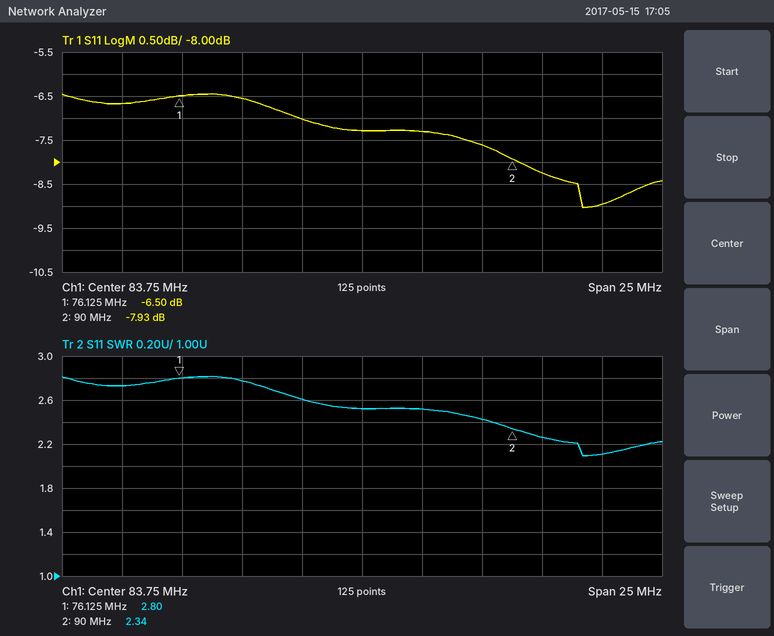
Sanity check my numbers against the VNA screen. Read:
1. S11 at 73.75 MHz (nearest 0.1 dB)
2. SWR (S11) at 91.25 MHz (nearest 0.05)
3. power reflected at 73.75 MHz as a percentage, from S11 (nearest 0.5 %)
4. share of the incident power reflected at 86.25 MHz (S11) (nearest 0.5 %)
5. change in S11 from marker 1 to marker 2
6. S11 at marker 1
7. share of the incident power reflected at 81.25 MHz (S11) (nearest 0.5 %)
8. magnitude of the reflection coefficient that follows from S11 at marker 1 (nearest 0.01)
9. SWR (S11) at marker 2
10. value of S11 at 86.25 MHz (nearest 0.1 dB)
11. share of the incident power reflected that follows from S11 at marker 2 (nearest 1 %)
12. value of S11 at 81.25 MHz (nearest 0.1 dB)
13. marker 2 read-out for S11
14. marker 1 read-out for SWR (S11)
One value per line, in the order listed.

-6.7 dB
2.25
21.5 %
18.5 %
-1.43 dB
-6.50 dB
20.0 %
0.47
2.34
-7.3 dB
16 %
-7.0 dB
-7.93 dB
2.80
